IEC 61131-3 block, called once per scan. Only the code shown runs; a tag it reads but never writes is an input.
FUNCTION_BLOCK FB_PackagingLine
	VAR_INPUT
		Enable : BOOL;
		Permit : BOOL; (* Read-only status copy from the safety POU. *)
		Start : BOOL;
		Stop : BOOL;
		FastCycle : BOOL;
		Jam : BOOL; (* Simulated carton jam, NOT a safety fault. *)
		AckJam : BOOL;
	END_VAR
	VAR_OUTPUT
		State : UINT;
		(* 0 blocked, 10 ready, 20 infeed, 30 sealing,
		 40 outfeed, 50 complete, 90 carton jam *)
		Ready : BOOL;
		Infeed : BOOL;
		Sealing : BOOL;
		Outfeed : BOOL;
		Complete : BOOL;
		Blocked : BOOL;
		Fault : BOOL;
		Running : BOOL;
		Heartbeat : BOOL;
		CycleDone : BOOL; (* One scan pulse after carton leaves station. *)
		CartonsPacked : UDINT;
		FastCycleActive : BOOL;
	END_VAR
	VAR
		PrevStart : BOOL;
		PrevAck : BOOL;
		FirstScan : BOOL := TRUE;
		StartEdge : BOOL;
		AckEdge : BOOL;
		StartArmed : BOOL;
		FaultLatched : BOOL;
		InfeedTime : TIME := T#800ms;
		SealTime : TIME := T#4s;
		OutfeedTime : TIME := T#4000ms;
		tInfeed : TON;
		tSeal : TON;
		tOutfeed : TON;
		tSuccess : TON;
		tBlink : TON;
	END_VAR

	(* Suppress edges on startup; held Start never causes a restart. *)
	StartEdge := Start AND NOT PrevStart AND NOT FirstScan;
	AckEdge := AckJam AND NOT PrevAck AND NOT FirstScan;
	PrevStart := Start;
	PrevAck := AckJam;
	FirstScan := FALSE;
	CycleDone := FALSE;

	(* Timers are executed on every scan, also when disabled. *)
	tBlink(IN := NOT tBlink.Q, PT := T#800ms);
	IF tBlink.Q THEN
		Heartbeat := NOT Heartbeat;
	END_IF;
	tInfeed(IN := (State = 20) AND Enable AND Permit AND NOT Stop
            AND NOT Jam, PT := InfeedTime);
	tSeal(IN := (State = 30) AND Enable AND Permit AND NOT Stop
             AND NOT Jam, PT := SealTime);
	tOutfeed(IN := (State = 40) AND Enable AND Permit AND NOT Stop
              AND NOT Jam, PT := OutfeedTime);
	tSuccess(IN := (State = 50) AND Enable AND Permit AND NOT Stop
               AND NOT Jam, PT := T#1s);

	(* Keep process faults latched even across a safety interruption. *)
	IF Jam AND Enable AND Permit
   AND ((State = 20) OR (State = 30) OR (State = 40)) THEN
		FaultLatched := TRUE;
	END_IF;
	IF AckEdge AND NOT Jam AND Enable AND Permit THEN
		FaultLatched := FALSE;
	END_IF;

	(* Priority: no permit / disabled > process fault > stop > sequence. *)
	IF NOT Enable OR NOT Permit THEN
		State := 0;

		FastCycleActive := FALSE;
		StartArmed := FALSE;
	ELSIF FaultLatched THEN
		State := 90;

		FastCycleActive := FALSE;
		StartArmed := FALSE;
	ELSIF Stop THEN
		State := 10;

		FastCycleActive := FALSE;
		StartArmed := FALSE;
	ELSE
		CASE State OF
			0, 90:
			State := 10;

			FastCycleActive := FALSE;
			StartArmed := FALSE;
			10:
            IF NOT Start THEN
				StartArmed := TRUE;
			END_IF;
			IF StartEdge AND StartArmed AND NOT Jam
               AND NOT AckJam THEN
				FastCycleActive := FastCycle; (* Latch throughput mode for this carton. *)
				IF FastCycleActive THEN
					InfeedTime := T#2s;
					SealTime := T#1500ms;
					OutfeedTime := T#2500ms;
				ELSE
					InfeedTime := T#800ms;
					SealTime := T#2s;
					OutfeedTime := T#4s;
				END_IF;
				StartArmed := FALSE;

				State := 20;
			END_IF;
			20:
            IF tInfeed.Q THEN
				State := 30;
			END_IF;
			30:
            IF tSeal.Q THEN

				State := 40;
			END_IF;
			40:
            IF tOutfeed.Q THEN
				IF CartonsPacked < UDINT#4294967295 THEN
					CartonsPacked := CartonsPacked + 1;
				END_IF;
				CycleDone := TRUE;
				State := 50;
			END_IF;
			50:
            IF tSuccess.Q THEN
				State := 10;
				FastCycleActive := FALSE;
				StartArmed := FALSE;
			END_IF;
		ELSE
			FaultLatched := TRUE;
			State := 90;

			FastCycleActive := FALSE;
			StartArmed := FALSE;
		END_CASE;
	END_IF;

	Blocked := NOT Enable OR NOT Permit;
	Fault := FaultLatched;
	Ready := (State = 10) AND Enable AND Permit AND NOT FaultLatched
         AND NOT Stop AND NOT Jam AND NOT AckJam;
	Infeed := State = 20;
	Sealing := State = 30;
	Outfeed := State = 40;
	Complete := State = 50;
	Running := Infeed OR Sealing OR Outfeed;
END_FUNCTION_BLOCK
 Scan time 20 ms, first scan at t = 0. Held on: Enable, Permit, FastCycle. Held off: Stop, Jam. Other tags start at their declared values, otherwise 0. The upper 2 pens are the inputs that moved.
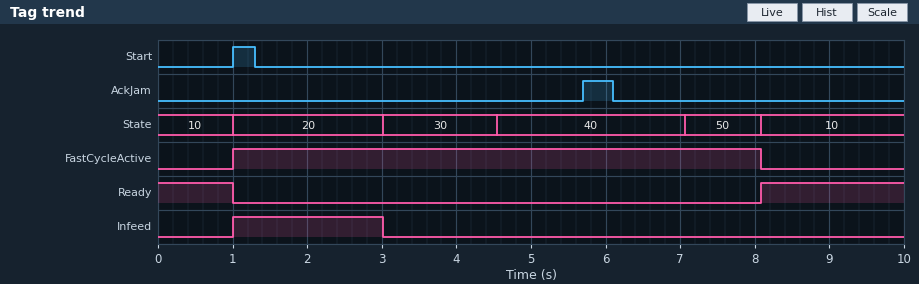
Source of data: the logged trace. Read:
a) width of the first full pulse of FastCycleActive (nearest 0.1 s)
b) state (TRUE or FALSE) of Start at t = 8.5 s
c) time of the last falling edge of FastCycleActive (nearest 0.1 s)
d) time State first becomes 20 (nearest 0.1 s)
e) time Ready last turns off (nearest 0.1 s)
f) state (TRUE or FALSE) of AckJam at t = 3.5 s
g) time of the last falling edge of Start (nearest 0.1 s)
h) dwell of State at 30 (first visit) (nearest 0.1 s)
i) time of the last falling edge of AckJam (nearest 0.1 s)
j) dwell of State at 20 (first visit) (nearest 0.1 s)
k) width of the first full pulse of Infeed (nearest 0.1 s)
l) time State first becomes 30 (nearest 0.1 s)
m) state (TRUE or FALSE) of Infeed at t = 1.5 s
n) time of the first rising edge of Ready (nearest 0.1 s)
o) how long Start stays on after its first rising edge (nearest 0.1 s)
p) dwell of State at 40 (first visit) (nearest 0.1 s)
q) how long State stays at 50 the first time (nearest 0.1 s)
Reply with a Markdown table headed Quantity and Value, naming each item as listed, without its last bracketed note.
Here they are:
| Quantity | Value |
|---|---|
| width of the first full pulse of FastCycleActive | 7.1 s |
| state (TRUE or FALSE) of Start at t = 8.5 s | FALSE |
| time of the last falling edge of FastCycleActive | 8.1 s |
| time State first becomes 20 | 1.0 s |
| time Ready last turns off | 1.0 s |
| state (TRUE or FALSE) of AckJam at t = 3.5 s | FALSE |
| time of the last falling edge of Start | 1.3 s |
| dwell of State at 30 (first visit) | 1.5 s |
| time of the last falling edge of AckJam | 6.1 s |
| dwell of State at 20 (first visit) | 2.0 s |
| width of the first full pulse of Infeed | 2.0 s |
| time State first becomes 30 | 3.0 s |
| state (TRUE or FALSE) of Infeed at t = 1.5 s | TRUE |
| time of the first rising edge of Ready | 8.1 s |
| how long Start stays on after its first rising edge | 0.3 s |
| dwell of State at 40 (first visit) | 2.5 s |
| how long State stays at 50 the first time | 1.0 s |
